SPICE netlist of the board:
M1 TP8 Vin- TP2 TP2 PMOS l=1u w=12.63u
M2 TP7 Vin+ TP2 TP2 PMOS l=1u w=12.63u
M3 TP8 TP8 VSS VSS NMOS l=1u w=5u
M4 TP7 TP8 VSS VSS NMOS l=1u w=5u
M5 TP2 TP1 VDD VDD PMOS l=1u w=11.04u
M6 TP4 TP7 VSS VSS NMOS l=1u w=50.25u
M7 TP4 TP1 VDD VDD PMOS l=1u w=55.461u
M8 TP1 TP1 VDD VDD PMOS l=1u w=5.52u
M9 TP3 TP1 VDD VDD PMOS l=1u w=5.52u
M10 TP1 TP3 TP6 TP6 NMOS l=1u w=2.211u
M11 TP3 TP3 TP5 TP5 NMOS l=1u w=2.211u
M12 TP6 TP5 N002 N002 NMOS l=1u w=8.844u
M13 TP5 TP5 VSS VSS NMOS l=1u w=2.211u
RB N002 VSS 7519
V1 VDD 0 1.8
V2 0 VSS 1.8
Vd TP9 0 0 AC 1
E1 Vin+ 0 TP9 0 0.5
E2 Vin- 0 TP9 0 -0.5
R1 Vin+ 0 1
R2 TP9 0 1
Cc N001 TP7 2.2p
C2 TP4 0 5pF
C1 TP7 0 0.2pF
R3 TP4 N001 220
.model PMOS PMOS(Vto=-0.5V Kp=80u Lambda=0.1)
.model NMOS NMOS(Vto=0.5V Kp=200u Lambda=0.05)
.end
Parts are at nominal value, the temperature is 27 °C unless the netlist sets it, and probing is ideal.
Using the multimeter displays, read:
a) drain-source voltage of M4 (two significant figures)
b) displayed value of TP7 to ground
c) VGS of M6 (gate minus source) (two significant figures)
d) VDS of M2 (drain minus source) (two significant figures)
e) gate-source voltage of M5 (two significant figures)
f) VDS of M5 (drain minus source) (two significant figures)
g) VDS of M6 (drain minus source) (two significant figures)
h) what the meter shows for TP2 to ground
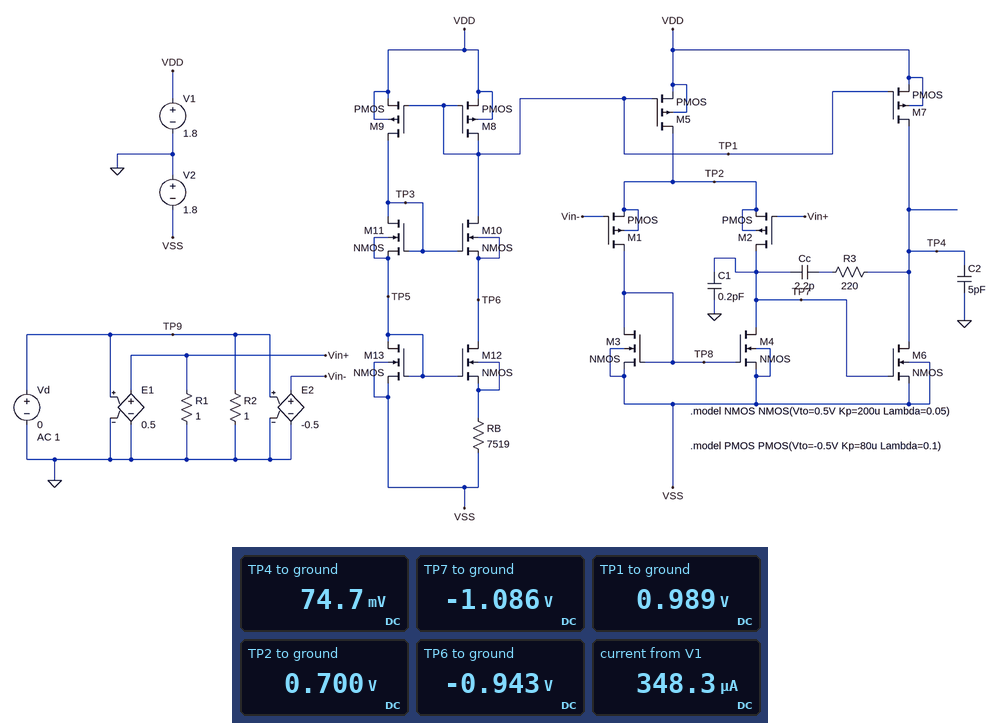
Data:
710 mV
-1.086 V
710 mV
-1.8 V
-810 mV
-1.1 V
1.9 V
0.700 V
